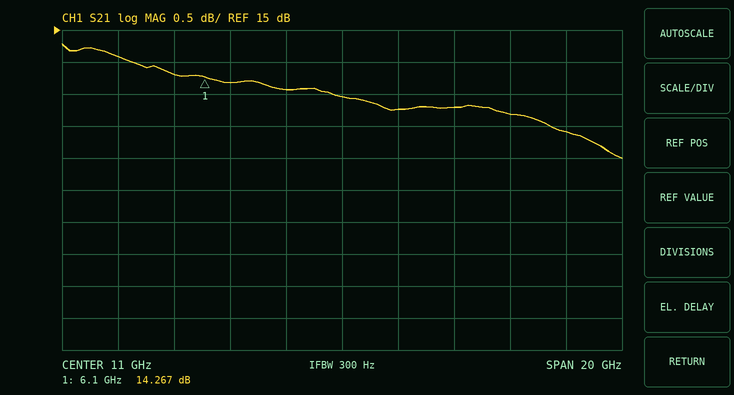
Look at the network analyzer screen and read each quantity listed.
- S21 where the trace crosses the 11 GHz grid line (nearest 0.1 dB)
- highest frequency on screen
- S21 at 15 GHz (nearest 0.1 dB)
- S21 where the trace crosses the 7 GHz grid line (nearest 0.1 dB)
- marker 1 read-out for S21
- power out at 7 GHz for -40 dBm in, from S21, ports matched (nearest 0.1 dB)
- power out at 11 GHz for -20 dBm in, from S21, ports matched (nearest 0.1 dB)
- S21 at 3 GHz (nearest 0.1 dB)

14.0 dB
21 GHz
13.8 dB
14.2 dB
14.267 dB
-25.8 dBm
-6.0 dBm
14.6 dB
